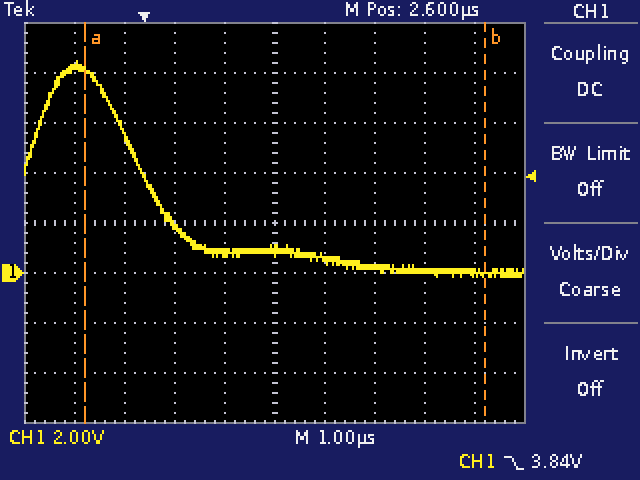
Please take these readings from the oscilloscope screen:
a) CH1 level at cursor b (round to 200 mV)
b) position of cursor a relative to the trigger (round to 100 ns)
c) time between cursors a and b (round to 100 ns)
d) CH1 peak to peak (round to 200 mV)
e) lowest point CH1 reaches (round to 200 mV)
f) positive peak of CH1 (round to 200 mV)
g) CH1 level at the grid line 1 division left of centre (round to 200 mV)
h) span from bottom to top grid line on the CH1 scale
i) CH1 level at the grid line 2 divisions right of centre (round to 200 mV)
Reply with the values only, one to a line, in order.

0.0 V
-1.2 µs
8.0 µs
8.6 V
-200 mV
8.4 V
800 mV
16 V
200 mV
